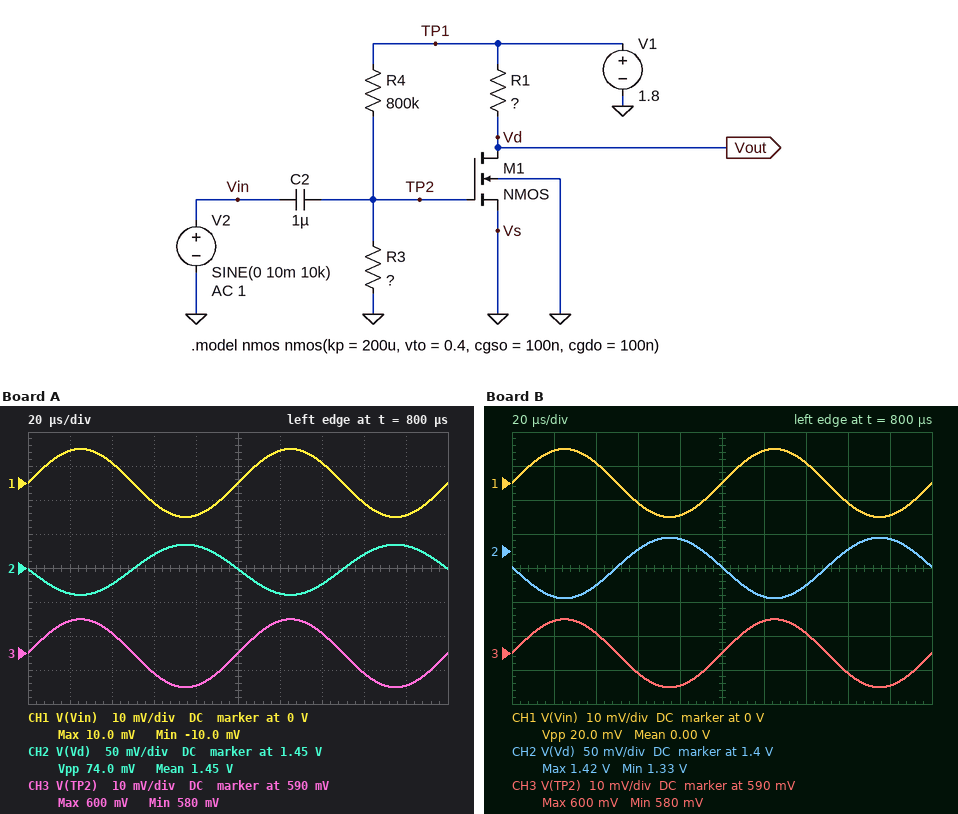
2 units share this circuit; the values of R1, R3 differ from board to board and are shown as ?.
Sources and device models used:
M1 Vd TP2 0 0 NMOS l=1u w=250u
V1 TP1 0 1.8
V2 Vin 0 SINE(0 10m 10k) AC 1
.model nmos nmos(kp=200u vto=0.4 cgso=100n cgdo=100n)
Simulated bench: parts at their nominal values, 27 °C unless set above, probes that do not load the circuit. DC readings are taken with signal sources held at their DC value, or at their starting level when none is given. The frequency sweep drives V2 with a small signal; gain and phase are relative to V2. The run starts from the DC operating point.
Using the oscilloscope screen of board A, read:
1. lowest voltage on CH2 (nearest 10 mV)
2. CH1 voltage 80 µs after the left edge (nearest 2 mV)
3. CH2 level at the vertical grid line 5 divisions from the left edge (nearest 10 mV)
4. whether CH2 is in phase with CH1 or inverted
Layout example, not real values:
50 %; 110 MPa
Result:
1.41 V; -10 mV; 1.45 V; inverted
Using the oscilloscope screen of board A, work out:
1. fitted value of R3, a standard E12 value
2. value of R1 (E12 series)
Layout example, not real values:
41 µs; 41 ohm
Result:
390 kΩ; 390 Ω
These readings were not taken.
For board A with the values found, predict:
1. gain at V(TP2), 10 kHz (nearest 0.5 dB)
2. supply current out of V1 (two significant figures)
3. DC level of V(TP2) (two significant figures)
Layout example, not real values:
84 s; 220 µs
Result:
0 dB; 900 µA; 590 mV
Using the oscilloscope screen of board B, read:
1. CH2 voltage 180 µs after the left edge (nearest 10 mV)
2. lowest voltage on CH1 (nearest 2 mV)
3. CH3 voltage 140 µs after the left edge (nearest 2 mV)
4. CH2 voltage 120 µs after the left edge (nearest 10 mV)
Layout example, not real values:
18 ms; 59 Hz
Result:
1.42 V; -10 mV; 596 mV; 1.33 V
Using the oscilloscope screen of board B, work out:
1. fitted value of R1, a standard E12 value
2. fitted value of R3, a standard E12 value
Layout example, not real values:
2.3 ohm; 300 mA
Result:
470 Ω; 390 kΩ
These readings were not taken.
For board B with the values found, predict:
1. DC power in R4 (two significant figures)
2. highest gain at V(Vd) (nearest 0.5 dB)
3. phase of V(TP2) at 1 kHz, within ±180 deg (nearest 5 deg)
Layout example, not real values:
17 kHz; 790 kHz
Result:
1.8 µW; 13.0 dB; 0 deg
